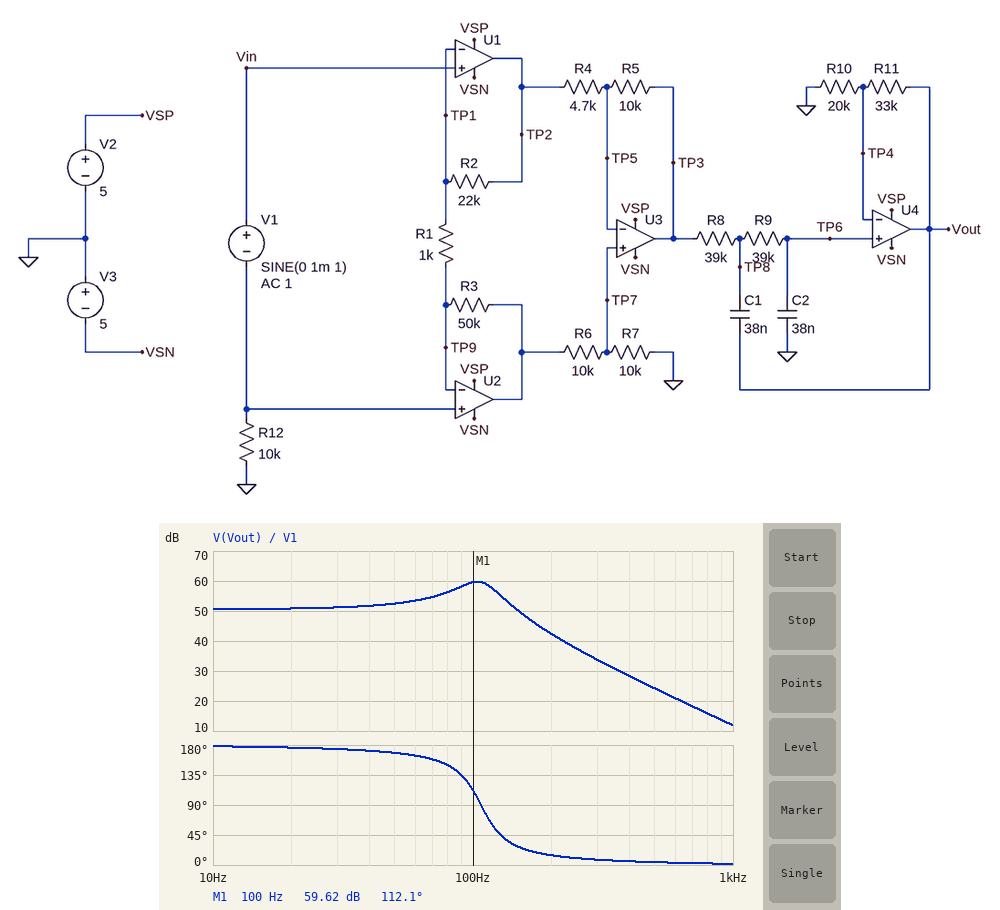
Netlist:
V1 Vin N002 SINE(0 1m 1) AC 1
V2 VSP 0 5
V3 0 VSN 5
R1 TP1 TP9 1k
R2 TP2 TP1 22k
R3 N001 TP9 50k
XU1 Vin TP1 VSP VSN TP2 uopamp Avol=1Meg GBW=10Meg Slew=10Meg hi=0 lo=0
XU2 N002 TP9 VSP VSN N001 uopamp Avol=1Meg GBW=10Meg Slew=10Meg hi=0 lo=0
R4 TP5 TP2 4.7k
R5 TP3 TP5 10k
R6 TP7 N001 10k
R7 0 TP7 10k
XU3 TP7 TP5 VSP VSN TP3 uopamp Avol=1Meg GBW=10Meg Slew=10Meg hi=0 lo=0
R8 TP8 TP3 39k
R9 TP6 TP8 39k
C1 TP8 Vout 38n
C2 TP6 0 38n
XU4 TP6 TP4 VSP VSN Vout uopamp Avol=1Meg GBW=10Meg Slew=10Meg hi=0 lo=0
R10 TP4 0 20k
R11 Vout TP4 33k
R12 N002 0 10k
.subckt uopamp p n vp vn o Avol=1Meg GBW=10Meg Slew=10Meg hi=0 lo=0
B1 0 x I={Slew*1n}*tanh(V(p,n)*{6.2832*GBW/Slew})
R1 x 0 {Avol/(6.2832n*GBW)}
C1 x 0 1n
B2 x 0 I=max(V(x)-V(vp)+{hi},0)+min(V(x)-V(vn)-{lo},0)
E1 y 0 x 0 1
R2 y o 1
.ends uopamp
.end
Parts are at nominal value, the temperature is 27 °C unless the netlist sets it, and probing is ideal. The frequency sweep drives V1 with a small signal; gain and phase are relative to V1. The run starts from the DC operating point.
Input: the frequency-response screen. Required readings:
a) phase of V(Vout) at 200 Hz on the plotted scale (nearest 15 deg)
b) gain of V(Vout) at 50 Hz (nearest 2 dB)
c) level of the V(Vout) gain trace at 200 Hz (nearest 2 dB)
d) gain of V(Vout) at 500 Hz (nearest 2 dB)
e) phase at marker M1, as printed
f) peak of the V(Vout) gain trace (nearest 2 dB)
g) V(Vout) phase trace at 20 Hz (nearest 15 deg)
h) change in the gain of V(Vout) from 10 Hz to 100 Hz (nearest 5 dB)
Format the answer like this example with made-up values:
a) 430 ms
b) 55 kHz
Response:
a) 15 deg
b) 52 dB
c) 42 dB
d) 24 dB
e) 112.1 deg
f) 60 dB
g) 180 deg
h) 10 dB
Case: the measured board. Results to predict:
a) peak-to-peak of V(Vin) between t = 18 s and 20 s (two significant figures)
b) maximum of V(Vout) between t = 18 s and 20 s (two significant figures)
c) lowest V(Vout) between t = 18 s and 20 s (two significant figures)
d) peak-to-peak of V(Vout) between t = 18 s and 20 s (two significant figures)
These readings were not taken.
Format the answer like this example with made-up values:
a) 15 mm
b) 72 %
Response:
a) 2.0 mV
b) 340 mV
c) -340 mV
d) 670 mV
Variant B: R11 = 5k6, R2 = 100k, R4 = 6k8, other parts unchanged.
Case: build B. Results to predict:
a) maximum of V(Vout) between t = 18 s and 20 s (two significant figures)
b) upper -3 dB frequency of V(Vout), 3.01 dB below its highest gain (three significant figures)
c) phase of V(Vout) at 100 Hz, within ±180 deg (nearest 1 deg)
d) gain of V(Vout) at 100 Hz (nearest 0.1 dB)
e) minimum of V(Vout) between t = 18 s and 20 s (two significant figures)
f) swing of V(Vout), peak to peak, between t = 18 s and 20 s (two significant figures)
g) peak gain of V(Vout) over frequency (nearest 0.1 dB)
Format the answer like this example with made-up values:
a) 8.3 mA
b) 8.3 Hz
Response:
a) 270 mV
b) 85.2 Hz
c) 95 deg
d) 44.5 dB
e) -270 mV
f) 540 mV
g) 48.6 dB
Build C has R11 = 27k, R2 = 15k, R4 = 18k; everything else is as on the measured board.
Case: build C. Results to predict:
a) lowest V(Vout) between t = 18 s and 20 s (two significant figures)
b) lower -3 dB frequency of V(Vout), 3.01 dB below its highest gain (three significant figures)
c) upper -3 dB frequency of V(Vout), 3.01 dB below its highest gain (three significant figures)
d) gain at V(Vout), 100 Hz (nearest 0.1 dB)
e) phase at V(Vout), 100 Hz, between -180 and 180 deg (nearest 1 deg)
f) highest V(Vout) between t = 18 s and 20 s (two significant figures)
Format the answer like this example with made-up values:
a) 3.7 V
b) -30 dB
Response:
a) -110 mV
b) 44.8 Hz
c) 127 Hz
d) 45.2 dB
e) 102 deg
f) 110 mV
